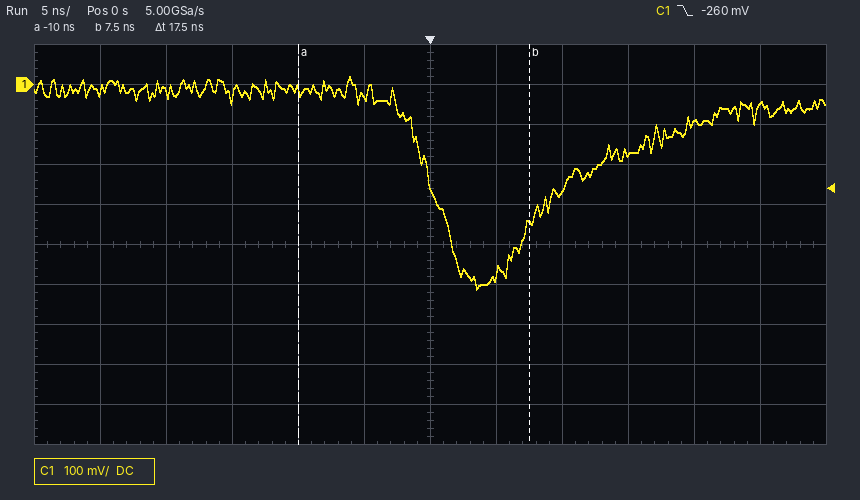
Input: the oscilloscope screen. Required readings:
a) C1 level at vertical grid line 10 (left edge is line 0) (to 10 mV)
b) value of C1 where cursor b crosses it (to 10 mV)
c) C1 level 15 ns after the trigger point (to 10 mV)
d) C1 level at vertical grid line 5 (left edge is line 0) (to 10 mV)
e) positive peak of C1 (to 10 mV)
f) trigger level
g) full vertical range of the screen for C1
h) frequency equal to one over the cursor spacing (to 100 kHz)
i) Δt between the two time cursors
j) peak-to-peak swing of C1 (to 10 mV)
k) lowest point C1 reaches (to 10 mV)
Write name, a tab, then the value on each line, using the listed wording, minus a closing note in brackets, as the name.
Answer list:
C1 level at vertical grid line 10 (left edge is line 0)	-100 mV
value of C1 where cursor b crosses it	-350 mV
C1 level 15 ns after the trigger point	-170 mV
C1 level at vertical grid line 5 (left edge is line 0)	-30 mV
positive peak of C1	20 mV
trigger level	-260 mV
full vertical range of the screen for C1	1 V
frequency equal to one over the cursor spacing	57.1 MHz
Δt between the two time cursors	17.5 ns
peak-to-peak swing of C1	530 mV
lowest point C1 reaches	-510 mV
